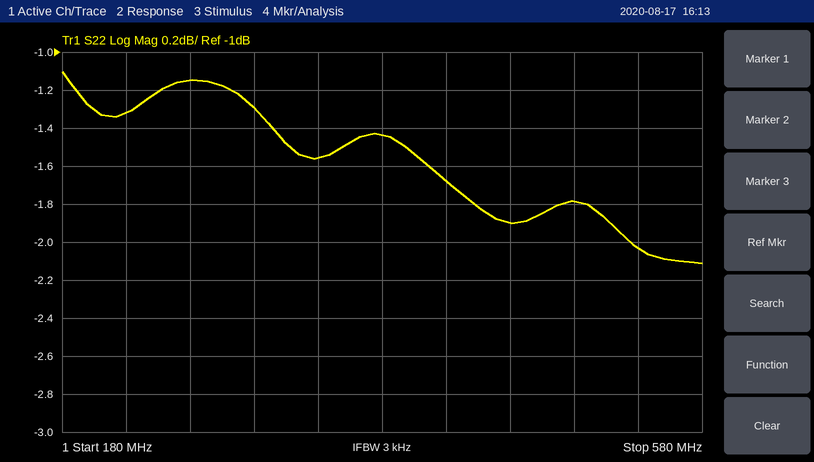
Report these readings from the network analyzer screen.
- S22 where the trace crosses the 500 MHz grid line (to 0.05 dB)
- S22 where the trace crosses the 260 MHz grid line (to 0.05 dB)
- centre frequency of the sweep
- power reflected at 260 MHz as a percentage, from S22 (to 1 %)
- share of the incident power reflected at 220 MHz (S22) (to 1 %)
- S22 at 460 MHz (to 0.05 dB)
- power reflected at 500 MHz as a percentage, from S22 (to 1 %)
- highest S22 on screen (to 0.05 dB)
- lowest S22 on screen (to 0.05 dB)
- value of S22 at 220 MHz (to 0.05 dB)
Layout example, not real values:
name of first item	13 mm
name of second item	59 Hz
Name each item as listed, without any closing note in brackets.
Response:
S22 where the trace crosses the 500 MHz grid line	-1.80 dB
S22 where the trace crosses the 260 MHz grid line	-1.15 dB
centre frequency of the sweep	380 MHz
power reflected at 260 MHz as a percentage, from S22	77 %
share of the incident power reflected at 220 MHz (S22)	74 %
S22 at 460 MHz	-1.90 dB
power reflected at 500 MHz as a percentage, from S22	66 %
highest S22 on screen	-1.10 dB
lowest S22 on screen	-2.10 dB
value of S22 at 220 MHz	-1.30 dB
